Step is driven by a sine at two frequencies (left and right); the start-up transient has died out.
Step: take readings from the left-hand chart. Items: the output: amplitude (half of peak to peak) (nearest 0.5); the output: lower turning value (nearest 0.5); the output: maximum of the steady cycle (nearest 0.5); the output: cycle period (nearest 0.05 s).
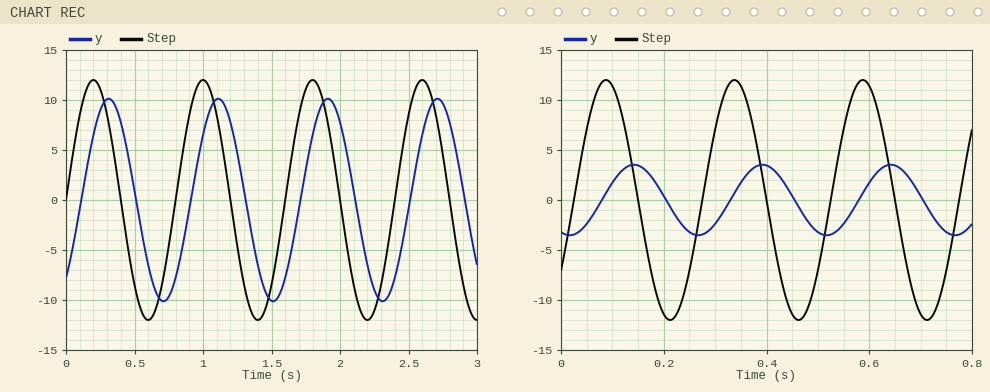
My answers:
10.0
-10.0
10.0
0.80 s
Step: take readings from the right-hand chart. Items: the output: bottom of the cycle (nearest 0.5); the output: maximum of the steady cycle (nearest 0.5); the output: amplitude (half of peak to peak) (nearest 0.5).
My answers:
-3.5
3.5
3.5
